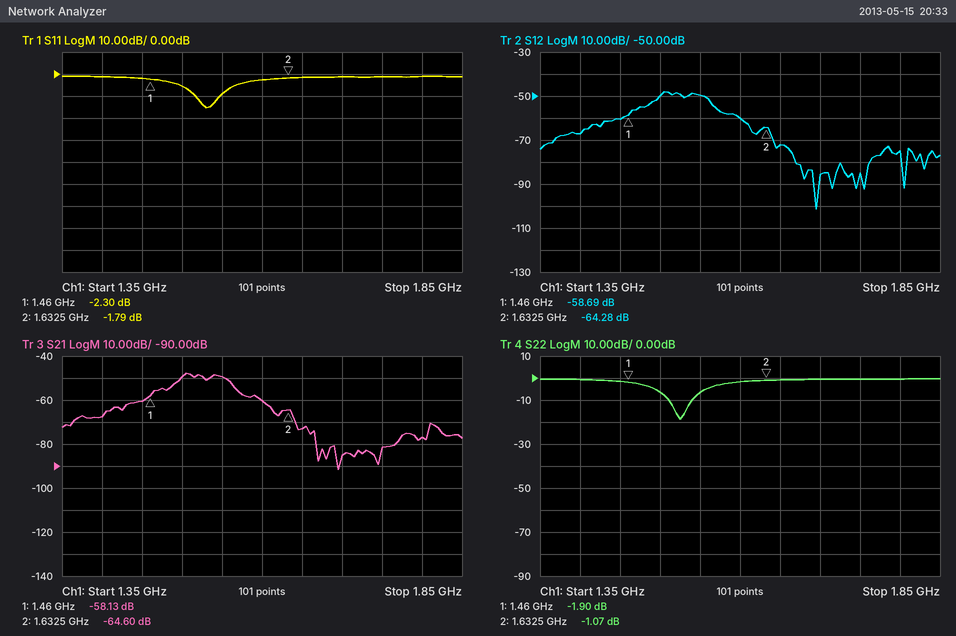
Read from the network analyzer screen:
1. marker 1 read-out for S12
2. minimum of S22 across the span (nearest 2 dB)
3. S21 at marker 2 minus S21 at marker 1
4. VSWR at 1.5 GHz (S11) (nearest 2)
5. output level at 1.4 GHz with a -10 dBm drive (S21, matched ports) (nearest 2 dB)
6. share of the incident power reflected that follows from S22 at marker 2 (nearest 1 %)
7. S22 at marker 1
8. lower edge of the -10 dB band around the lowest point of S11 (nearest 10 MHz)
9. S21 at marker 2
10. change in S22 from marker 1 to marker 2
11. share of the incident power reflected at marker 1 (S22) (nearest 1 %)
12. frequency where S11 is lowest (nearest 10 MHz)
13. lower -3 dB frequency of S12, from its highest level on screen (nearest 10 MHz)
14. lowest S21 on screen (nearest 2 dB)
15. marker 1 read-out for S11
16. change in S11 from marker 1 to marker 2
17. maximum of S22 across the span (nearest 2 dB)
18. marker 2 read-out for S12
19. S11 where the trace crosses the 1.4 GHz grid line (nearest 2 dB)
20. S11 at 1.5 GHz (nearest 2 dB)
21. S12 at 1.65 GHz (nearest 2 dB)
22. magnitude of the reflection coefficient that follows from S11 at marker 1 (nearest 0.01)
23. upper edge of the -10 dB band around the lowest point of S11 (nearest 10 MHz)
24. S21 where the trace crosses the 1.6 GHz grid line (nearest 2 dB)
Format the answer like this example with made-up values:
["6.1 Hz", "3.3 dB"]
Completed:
["-58.69 dB", "-18 dB", "-6.47 dB", "4", "-78 dBm", "78 %", "-1.90 dB", "1.52 GHz", "-64.60 dB", "0.83 dB", "65 %", "1.53 GHz", "1.50 GHz", "-92 dB", "-2.30 dB", "0.51 dB", "0 dB", "-64.28 dB", "-2 dB", "-6 dB", "-72 dB", "0.77", "1.55 GHz", "-60 dB"]
